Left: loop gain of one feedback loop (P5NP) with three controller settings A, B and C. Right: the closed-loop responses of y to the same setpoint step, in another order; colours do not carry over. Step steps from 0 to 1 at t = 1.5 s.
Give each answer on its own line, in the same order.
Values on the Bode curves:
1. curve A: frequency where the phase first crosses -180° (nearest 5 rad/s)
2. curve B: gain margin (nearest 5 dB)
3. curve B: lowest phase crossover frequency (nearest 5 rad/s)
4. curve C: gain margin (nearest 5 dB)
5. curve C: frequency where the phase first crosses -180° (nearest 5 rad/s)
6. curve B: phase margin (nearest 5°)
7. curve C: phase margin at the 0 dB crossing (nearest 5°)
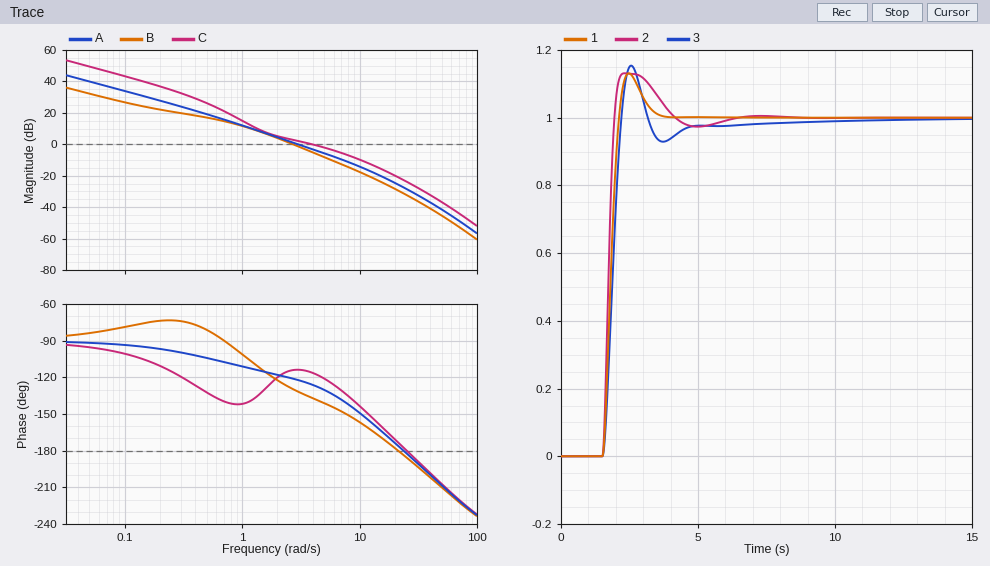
25 rad/s
30 dB
20 rad/s
25 dB
25 rad/s
50°
65°
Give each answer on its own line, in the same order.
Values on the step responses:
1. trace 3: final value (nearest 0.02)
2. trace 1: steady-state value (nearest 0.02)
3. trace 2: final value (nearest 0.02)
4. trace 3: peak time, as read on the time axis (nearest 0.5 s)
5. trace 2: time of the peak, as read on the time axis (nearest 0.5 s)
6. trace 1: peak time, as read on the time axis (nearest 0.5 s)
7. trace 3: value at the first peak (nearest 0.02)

1.00
1.00
1.00
2.5 s
2.5 s
2.5 s
1.16
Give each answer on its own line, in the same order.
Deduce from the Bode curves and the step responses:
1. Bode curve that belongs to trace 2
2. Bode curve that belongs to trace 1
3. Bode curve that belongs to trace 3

C
A
B
